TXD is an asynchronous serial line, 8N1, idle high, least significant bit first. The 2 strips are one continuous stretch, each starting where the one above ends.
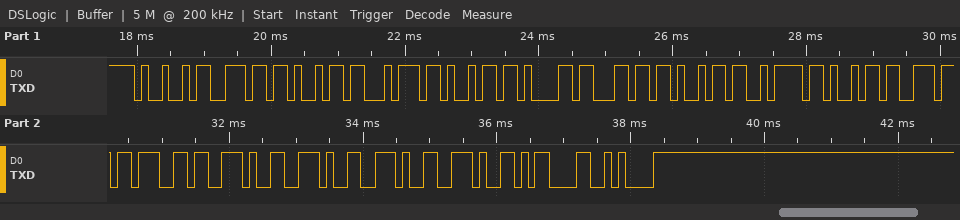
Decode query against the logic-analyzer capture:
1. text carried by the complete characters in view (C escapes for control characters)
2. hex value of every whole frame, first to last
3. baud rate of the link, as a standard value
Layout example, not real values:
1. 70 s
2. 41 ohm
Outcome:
1. "Initializing....\r\n"
2. 49 6E 69 74 69 61 6C 69 7A 69 6E 67 2E 2E 2E 2E 0D 0A
3. 9600 baud
